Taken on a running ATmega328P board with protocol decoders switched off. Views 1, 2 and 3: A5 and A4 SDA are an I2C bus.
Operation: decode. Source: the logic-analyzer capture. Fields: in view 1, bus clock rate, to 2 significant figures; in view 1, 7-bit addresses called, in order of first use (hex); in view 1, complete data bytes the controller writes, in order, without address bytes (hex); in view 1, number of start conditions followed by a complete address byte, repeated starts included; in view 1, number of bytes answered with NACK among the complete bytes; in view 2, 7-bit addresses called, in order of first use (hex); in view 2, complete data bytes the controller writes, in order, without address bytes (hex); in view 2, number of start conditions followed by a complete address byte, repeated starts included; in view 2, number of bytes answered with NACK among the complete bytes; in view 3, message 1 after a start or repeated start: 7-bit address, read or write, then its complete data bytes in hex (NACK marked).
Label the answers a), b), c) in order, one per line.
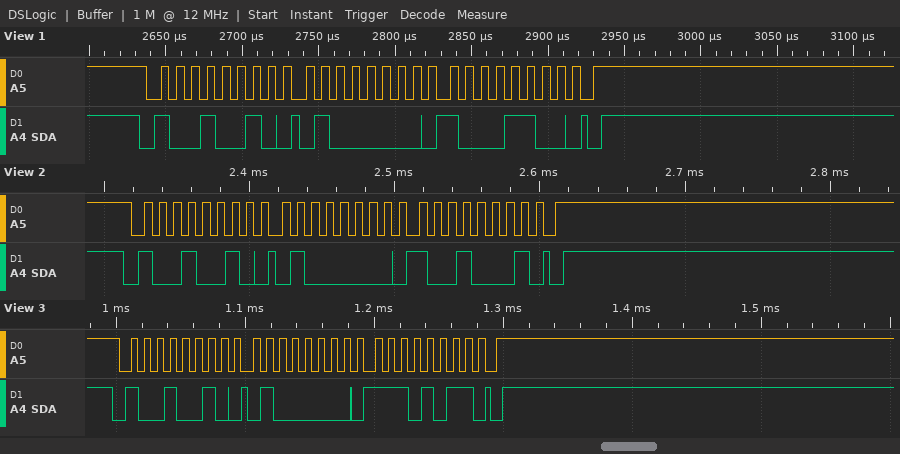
a) 100 kHz
b) 0x49
c) 40 8C
d) 1
e) 0
f) 0x49
g) 40 91
h) 1
i) 0
j) 0x49 write: 40 EB
